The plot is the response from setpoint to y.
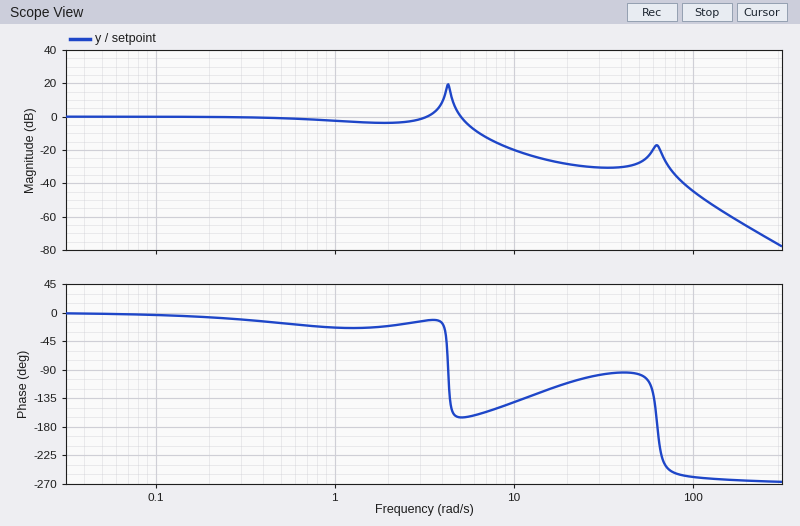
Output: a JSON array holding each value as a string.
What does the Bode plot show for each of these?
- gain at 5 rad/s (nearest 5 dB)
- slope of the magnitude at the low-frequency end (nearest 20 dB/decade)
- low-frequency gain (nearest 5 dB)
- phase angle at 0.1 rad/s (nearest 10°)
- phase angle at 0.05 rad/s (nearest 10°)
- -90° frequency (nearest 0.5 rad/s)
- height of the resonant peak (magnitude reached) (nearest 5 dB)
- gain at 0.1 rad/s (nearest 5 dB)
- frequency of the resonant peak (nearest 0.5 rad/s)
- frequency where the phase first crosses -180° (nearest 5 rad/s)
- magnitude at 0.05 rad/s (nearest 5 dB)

["0 dB", "0 dB/decade", "0 dB", "0°", "0°", "4.5 rad/s", "20 dB", "0 dB", "4.5 rad/s", "65 rad/s", "0 dB"]
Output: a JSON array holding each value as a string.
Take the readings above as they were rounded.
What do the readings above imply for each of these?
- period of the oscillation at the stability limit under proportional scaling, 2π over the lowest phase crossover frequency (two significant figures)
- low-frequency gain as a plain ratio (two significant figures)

["0.097 s", "1.0"]
